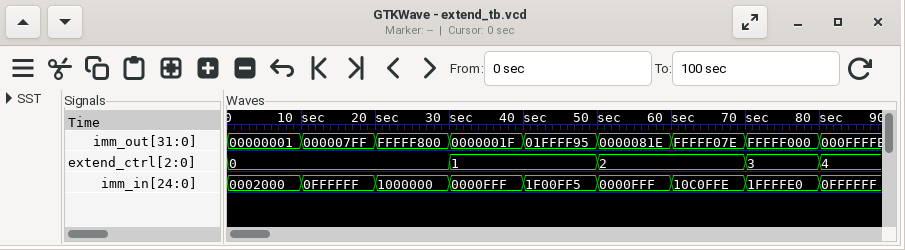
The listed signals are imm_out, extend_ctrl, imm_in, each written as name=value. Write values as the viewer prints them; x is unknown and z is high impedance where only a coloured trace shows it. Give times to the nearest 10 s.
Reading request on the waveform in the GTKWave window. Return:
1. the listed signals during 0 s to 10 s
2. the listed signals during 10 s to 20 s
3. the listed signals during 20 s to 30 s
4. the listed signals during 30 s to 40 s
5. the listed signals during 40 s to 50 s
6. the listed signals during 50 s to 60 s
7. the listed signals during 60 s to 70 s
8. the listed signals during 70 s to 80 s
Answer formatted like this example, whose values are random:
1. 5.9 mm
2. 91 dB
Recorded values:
1. imm_out=00000001, extend_ctrl=0, imm_in=0002000
2. imm_out=000007FF, extend_ctrl=0, imm_in=0FFFFFF
3. imm_out=FFFFF800, extend_ctrl=0, imm_in=1000000
4. imm_out=0000001F, extend_ctrl=1, imm_in=0000FFF
5. imm_out=01FFFF95, extend_ctrl=1, imm_in=1F00FF5
6. imm_out=0000081E, extend_ctrl=2, imm_in=0000FFF
7. imm_out=FFFFF07E, extend_ctrl=2, imm_in=10C0FFE
8. imm_out=FFFFF000, extend_ctrl=3, imm_in=1FFFFE0
